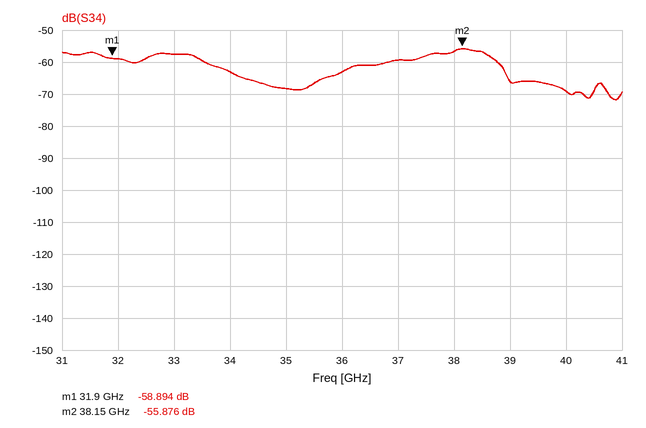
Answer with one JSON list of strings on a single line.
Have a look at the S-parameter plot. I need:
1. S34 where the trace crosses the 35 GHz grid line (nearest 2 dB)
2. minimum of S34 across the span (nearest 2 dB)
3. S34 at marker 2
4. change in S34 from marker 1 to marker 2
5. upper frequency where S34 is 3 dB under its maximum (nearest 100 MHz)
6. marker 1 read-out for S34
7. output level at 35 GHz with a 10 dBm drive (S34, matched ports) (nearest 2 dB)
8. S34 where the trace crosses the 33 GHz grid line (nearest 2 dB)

["-68 dB", "-72 dB", "-55.876 dB", "3.018 dB", "38.7 GHz", "-58.894 dB", "-58 dBm", "-58 dB"]
